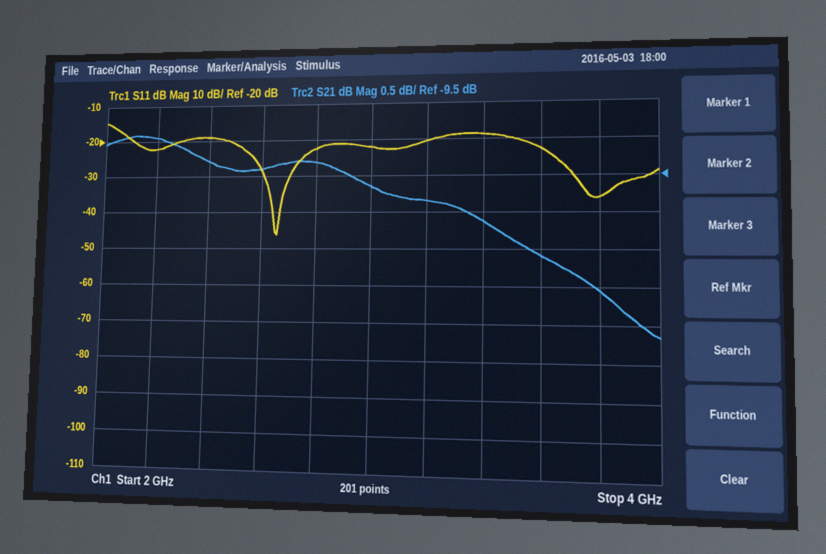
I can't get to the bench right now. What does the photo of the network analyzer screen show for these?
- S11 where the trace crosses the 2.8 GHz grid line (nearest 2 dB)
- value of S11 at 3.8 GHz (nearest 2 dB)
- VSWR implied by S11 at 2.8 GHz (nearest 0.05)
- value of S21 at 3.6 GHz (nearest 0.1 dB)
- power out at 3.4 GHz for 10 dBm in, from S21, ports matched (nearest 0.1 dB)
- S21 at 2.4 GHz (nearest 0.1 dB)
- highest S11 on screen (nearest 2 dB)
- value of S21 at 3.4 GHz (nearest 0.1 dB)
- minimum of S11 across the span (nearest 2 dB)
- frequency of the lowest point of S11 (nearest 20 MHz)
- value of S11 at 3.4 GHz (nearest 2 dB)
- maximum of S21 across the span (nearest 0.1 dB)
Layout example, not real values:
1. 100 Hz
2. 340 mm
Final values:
1. -22 dB
2. -36 dB
3. 1.15
4. -10.6 dB
5. -0.1 dBm
6. -9.3 dB
7. -14 dB
8. -10.1 dB
9. -46 dB
10. 2.66 GHz
11. -18 dB
12. -8.9 dB
